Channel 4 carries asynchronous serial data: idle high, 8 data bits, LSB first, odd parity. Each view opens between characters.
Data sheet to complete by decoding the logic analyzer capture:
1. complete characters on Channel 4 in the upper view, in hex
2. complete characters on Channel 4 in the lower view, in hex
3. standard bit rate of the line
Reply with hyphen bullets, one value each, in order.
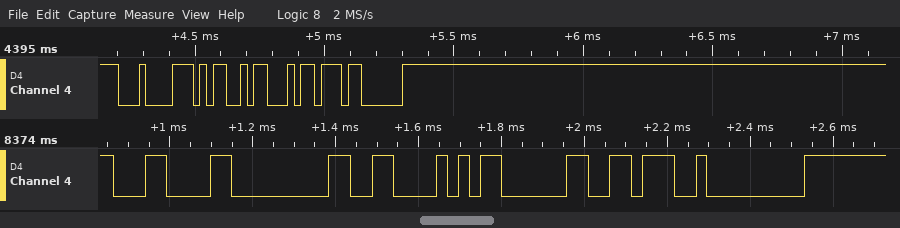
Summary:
- 84, 4D, B4, 03
- 0C, 00, 86, 03, 76, 00
- 38400 baud
